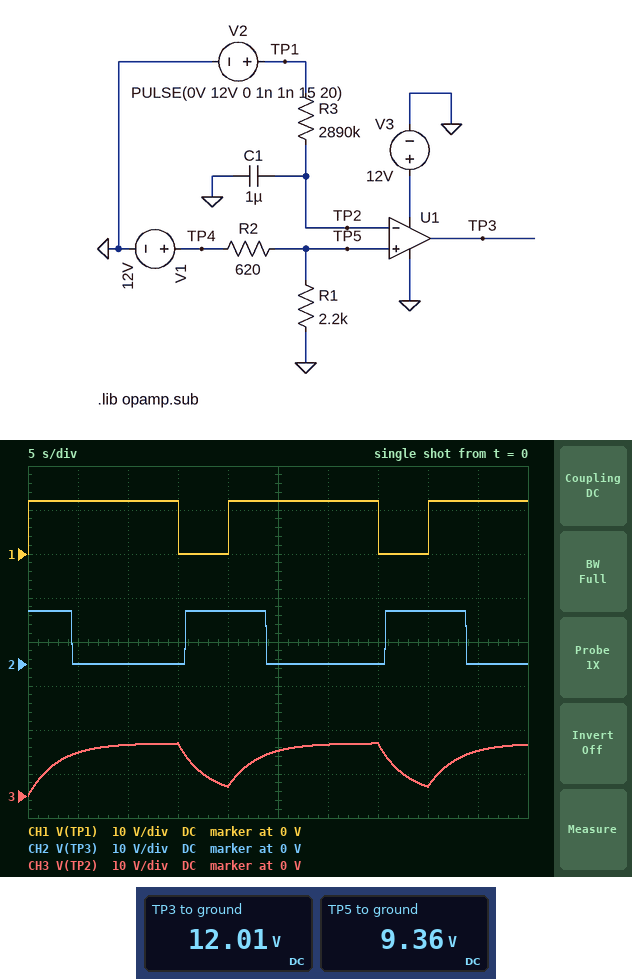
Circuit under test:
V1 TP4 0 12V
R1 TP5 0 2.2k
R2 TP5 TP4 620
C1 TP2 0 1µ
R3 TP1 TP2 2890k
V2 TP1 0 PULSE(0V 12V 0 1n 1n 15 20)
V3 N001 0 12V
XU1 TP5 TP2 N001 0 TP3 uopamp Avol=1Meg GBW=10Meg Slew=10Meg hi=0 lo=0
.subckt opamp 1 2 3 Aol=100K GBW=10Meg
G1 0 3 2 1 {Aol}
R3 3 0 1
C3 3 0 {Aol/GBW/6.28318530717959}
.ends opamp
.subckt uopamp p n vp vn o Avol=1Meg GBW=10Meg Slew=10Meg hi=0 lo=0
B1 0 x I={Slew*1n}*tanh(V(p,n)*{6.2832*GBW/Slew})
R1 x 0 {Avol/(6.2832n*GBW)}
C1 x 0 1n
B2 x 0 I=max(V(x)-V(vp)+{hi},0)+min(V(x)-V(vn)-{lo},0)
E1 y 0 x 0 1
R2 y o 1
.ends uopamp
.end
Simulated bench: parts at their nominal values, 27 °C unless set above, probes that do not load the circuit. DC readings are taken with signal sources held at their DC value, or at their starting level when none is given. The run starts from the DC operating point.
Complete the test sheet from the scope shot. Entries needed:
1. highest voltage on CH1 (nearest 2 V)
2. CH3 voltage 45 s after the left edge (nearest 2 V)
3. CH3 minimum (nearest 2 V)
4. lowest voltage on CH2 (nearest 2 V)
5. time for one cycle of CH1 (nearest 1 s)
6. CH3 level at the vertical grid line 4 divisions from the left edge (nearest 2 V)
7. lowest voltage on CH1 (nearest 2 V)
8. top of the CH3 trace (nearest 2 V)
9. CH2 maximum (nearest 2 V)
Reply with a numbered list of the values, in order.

1. 12 V
2. 10 V
3. 0 V
4. 0 V
5. 20 s
6. 2 V
7. 0 V
8. 12 V
9. 12 V
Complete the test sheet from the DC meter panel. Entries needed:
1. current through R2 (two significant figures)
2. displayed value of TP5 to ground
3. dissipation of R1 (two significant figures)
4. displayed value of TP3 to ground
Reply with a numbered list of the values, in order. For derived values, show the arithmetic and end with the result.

1. (12 V - 9.36 V) / 620 Ω = 4.3 mA
2. 9.36 V
3. (9.36 V)^2 / 2.2 kΩ = 40 mW
4. 12.01 V
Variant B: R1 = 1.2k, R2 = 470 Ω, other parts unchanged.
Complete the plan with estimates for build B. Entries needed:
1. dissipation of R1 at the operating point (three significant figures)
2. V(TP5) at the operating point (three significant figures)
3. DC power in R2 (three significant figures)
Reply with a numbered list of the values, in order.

1. 62.0 mW
2. 8.62 V
3. 24.3 mW
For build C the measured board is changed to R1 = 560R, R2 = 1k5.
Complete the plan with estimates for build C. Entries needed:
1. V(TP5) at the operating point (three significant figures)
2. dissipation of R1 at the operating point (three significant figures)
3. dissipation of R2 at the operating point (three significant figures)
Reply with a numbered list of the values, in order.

1. 3.26 V
2. 19.0 mW
3. 50.9 mW
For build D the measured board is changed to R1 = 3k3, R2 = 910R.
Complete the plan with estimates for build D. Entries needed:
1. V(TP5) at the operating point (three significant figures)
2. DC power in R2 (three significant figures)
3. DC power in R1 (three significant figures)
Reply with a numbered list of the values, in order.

1. 9.41 V
2. 7.39 mW
3. 26.8 mW
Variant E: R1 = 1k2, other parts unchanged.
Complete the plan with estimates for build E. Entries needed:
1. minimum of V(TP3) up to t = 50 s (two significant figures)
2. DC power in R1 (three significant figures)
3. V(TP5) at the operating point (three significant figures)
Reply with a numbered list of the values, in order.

1. -10 mV
2. 52.2 mW
3. 7.91 V
